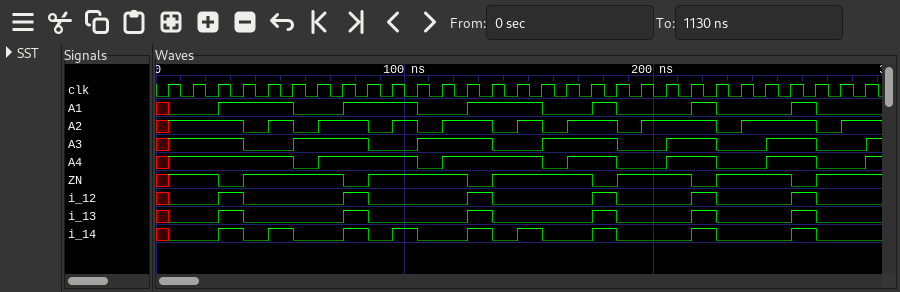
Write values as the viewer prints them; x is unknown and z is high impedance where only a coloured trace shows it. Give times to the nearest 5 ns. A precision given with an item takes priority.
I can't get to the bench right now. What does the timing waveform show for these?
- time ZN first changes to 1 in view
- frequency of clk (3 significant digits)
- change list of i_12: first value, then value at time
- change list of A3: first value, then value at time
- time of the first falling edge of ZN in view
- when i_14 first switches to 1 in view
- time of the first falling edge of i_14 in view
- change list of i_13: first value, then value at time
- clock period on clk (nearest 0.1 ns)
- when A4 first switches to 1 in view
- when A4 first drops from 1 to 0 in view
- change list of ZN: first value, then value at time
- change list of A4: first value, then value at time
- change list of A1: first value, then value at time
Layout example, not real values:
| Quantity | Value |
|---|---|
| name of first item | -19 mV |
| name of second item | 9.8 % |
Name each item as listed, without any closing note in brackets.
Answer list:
| Quantity | Value |
|---|---|
| time ZN first changes to 1 in view | 5 ns |
| frequency of clk | 100 MHz |
| change list of i_12: first value, then value at time | x, 0 at 5 ns, 1 at 25 ns, 0 at 35 ns, 1 at 75 ns, 0 at 85 ns, 1 at 125 ns, 0 at 135 ns, 1 at 175 ns, 0 at 185 ns, 1 at 215 ns, 0 at 225 ns, 1 at 255 ns, 0 at 265 ns |
| change list of A3: first value, then value at time | x, 1 at 5 ns, 0 at 35 ns, 1 at 55 ns, 0 at 85 ns, 1 at 105 ns, 0 at 135 ns, 1 at 155 ns, 0 at 185 ns, 1 at 205 ns, 0 at 225 ns, 1 at 245 ns, 0 at 265 ns, 1 at 285 ns |
| time of the first falling edge of ZN in view | 25 ns |
| when i_14 first switches to 1 in view | 25 ns |
| time of the first falling edge of i_14 in view | 35 ns |
| change list of i_13: first value, then value at time | x, 0 at 5 ns, 1 at 25 ns, 0 at 35 ns, 1 at 75 ns, 0 at 85 ns, 1 at 125 ns, 0 at 135 ns, 1 at 175 ns, 0 at 185 ns, 1 at 215 ns, 0 at 225 ns, 1 at 255 ns, 0 at 265 ns |
| clock period on clk | 10 ns |
| when A4 first switches to 1 in view | 5 ns |
| when A4 first drops from 1 to 0 in view | 55 ns |
| change list of ZN: first value, then value at time | x, 1 at 5 ns, 0 at 25 ns, 1 at 35 ns, 0 at 75 ns, 1 at 85 ns, 0 at 125 ns, 1 at 135 ns, 0 at 175 ns, 1 at 185 ns, 0 at 215 ns, 1 at 225 ns, 0 at 255 ns, 1 at 265 ns |
| change list of A4: first value, then value at time | x, 1 at 5 ns, 0 at 55 ns, 1 at 65 ns, 0 at 105 ns, 1 at 115 ns, 0 at 155 ns, 1 at 165 ns, 0 at 185 ns, 1 at 205 ns, 0 at 225 ns, 1 at 245 ns, 0 at 265 ns, 1 at 285 ns |
| change list of A1: first value, then value at time | x, 0 at 5 ns, 1 at 25 ns, 0 at 55 ns, 1 at 75 ns, 0 at 105 ns, 1 at 125 ns, 0 at 155 ns, 1 at 175 ns, 0 at 185 ns, 1 at 215 ns, 0 at 225 ns, 1 at 255 ns, 0 at 265 ns |
